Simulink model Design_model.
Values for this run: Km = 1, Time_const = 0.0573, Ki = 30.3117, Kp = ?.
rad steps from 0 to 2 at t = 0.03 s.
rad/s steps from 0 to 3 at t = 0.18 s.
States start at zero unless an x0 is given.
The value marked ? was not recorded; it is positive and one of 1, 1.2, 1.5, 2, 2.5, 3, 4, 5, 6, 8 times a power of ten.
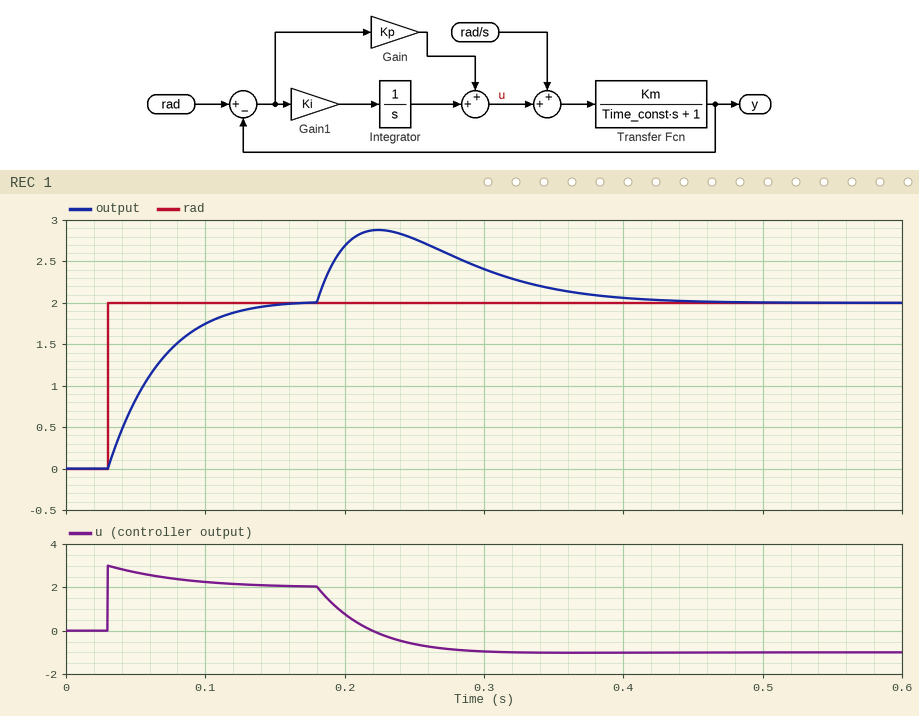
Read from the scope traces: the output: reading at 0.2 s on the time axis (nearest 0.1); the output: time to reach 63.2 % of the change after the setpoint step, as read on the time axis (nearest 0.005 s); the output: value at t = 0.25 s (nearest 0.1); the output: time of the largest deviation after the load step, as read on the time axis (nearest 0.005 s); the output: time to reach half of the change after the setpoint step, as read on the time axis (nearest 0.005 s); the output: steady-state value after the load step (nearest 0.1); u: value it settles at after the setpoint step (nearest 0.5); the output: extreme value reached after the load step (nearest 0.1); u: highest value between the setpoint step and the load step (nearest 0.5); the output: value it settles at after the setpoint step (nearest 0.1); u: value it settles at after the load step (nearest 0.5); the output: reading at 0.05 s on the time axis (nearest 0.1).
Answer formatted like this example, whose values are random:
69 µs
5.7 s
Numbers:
2.7
0.065 s
2.8
0.225 s
0.055 s
2.0
2.0
2.9
3.0
2.0
-1.0
0.8
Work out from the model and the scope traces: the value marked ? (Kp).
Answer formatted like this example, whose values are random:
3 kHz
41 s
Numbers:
1.5
